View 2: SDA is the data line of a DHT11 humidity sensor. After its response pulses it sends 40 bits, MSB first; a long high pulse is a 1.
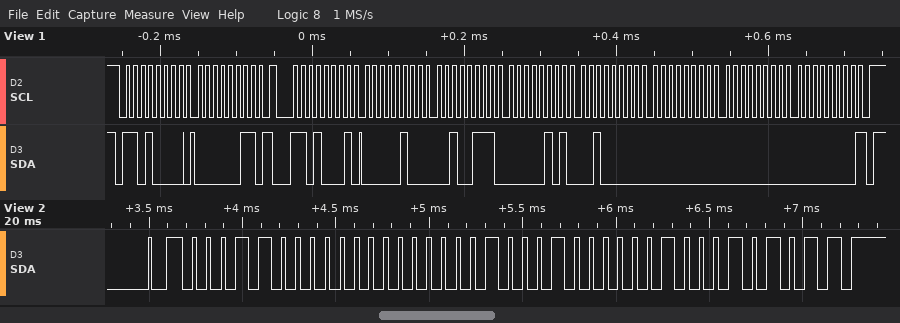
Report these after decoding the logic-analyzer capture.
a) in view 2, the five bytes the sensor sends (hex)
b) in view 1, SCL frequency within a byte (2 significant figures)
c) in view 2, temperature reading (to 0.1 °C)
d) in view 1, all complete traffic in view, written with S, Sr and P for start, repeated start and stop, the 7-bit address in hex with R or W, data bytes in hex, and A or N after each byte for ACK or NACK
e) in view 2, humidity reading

18 00 11 02 2B
100 kHz
17.2 °C
S 68W A 03 A Sr 68R A 04 A 27 A 05 A 20 A 00 A 00 A 00 N P
24 %
